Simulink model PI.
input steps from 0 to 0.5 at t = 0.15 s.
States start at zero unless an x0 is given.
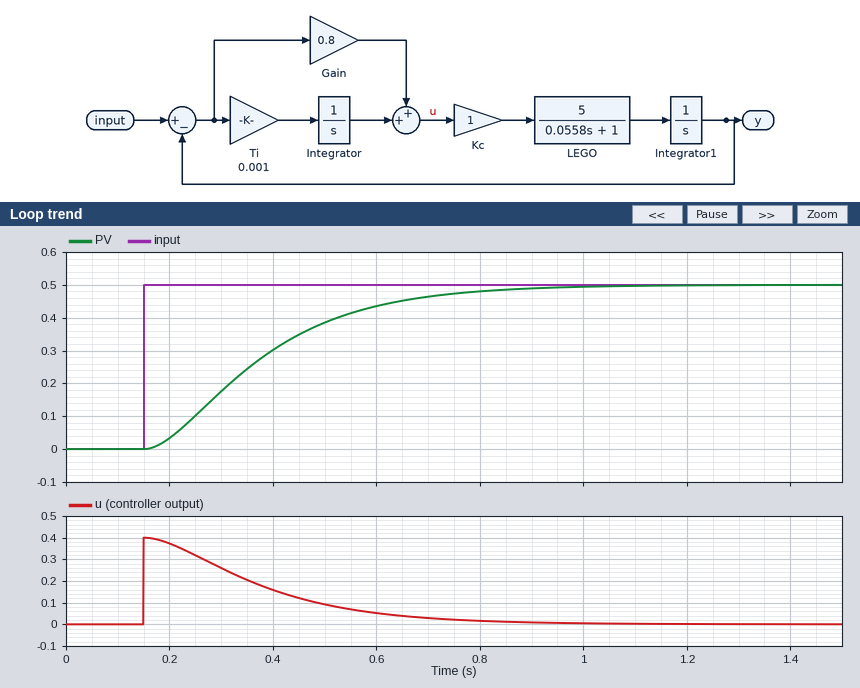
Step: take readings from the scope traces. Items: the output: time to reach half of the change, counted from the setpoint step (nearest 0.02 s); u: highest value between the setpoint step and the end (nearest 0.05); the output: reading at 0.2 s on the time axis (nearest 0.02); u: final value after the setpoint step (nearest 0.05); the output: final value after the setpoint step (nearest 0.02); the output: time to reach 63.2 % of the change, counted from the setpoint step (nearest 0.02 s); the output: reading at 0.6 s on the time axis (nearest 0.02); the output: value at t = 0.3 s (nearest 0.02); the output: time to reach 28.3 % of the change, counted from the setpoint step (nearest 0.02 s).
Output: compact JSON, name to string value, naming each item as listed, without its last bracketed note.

{"the output: time to reach half of the change, counted from the setpoint step": "0.20 s", "u: highest value between the setpoint step and the end": "0.40", "the output: reading at 0.2 s on the time axis": "0.04", "u: final value after the setpoint step": "0.00", "the output: final value after the setpoint step": "0.50", "the output: time to reach 63.2 % of the change, counted from the setpoint step": "0.26 s", "the output: reading at 0.6 s on the time axis": "0.44", "the output: value at t = 0.3 s": "0.18", "the output: time to reach 28.3 % of the change, counted from the setpoint step": "0.12 s"}
